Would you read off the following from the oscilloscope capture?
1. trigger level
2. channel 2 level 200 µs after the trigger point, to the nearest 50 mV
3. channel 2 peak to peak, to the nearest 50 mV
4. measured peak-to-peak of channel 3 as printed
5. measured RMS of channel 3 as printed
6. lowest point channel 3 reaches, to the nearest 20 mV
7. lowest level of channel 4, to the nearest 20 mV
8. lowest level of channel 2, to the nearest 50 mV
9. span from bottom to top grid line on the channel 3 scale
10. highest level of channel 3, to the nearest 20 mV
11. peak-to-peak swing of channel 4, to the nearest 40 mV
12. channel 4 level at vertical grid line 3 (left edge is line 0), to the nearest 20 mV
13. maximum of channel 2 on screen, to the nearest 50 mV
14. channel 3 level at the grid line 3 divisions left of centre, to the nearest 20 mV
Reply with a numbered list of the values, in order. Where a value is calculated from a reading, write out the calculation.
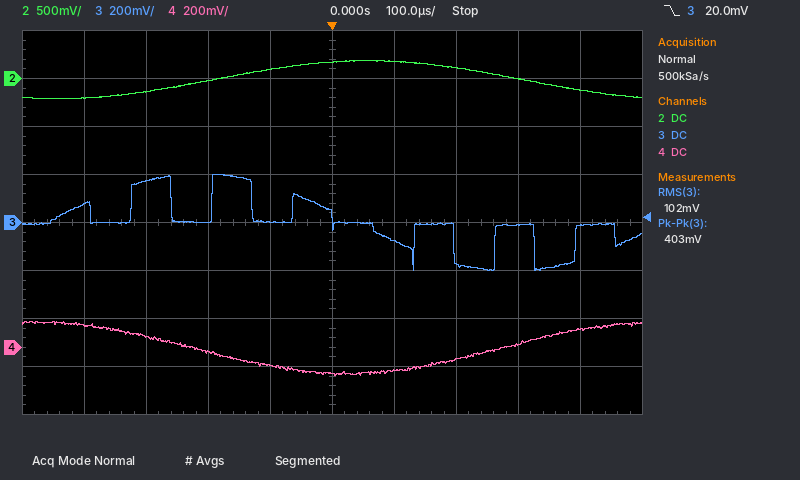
1. 20.0 mV
2. 100 mV
3. 200 mV − (-200 mV) = 400 mV
4. 403 mV
5. 102 mV
6. -200 mV
7. -120 mV
8. -200 mV
9. 1.6 V
10. 200 mV
11. 240 mV
12. -20 mV
13. 200 mV
14. 180 mV
